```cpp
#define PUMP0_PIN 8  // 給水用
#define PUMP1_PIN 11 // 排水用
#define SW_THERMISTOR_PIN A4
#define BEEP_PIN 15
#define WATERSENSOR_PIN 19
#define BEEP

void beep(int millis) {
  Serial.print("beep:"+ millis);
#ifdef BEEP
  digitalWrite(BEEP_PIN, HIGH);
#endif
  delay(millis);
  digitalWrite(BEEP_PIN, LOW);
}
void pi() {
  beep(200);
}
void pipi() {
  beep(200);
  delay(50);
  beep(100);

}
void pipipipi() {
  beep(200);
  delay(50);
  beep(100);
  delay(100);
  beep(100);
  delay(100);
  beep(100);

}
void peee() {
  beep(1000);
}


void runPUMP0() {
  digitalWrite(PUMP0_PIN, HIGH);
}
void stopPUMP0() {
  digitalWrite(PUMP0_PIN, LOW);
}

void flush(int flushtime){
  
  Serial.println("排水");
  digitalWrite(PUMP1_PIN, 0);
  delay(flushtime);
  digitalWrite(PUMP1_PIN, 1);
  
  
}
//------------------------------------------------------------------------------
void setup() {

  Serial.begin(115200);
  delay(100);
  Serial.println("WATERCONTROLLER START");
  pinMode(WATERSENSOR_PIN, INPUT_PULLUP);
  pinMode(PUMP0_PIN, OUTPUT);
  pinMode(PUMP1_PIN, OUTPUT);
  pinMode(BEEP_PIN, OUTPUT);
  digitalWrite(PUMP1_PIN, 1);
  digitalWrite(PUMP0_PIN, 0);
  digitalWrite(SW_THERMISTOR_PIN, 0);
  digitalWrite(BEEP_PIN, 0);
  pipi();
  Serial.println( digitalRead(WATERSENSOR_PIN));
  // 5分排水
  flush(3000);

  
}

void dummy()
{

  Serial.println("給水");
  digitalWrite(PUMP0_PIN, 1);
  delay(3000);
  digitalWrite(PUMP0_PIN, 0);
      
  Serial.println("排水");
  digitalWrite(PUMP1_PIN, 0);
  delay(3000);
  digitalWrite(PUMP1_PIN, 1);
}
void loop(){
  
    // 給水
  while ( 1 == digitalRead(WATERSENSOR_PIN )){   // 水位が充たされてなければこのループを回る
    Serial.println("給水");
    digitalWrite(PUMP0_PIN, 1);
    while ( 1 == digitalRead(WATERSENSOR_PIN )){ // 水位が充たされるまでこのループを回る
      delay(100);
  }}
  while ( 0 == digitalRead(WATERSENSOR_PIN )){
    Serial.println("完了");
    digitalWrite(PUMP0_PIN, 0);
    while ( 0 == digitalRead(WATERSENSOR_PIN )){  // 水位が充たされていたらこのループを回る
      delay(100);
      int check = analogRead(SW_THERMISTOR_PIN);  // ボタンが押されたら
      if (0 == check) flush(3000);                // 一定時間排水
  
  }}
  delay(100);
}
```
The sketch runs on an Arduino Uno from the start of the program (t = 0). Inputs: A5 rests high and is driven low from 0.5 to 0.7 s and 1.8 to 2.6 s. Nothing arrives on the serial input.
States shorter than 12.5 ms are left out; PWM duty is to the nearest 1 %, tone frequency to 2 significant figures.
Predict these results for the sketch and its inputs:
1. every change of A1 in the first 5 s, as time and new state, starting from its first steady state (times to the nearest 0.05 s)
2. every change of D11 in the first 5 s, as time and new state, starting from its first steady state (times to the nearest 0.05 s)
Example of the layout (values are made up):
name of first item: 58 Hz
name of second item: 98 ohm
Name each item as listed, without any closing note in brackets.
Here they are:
every change of A1 in the first 5 s, as time and new state, starting from its first steady state: 0.1 s high; 0.3 s low; 0.35 s high; 0.45 s low
every change of D11 in the first 5 s, as time and new state, starting from its first steady state: 0.1 s high; 0.45 s low; 3.45 s high
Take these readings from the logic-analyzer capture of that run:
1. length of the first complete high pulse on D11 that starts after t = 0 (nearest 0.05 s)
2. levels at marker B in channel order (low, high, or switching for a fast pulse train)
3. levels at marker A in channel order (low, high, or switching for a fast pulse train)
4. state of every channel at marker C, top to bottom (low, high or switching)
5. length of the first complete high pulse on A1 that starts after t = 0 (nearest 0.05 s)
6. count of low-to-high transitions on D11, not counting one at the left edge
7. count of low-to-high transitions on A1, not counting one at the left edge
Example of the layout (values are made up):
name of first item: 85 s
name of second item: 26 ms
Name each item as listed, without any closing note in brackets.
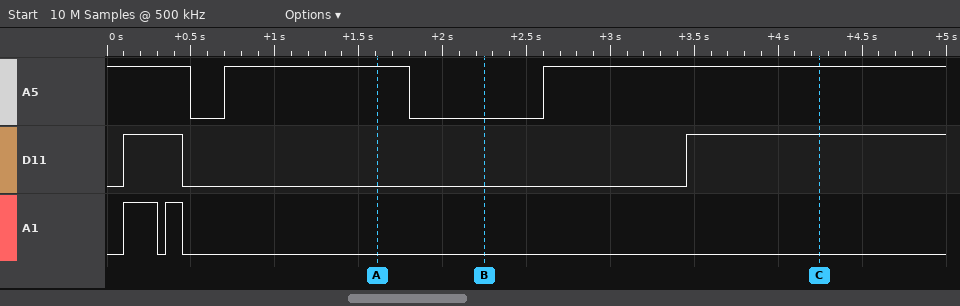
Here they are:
length of the first complete high pulse on D11 that starts after t = 0: 0.35 s
levels at marker B in channel order: A5 low, D11 low, A1 low
levels at marker A in channel order: A5 high, D11 low, A1 low
state of every channel at marker C, top to bottom: A5 high, D11 high, A1 low
length of the first complete high pulse on A1 that starts after t = 0: 0.20 s
count of low-to-high transitions on D11, not counting one at the left edge: 2
count of low-to-high transitions on A1, not counting one at the left edge: 2
